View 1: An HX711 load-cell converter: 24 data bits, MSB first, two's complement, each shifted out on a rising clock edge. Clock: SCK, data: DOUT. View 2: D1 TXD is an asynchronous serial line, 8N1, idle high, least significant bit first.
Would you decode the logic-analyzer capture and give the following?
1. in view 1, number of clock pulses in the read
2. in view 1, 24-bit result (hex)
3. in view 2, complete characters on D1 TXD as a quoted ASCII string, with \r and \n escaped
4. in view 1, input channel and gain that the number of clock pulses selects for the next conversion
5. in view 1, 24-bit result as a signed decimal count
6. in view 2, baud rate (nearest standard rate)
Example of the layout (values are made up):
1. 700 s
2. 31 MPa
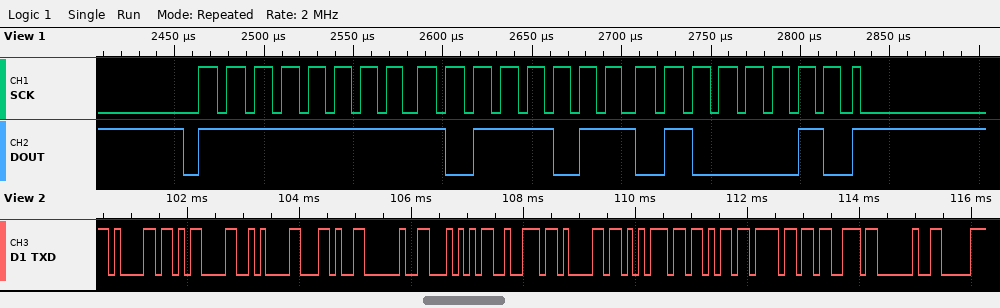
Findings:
1. 25
2. 0xFFBB42
3. "a\r\n, Traukos "
4. channel A, gain 128
5. -17598
6. 9600 baud
